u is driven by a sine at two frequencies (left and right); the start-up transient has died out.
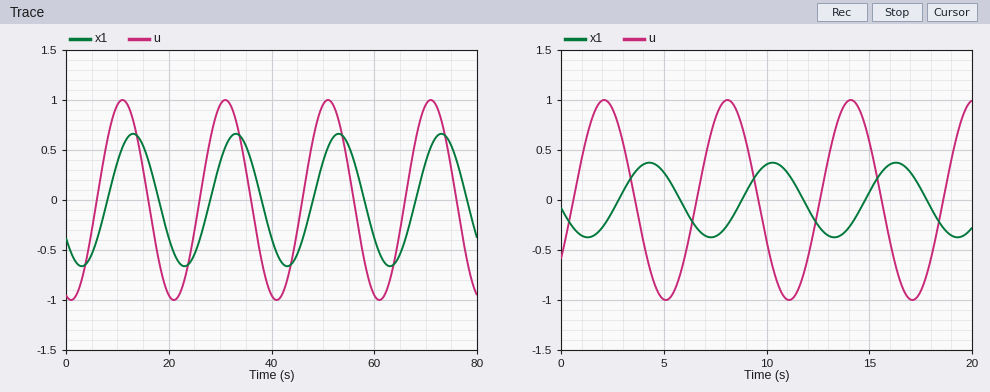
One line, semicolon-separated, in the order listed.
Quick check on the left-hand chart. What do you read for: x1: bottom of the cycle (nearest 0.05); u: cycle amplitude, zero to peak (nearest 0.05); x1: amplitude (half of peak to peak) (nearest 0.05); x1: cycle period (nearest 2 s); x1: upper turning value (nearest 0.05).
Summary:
-0.65; 1.00; 0.65; 20 s; 0.65
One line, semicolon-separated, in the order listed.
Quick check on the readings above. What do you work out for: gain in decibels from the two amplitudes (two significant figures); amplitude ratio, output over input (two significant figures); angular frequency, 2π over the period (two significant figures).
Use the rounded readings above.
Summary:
-3.7 dB; 0.65; 0.31 rad/s
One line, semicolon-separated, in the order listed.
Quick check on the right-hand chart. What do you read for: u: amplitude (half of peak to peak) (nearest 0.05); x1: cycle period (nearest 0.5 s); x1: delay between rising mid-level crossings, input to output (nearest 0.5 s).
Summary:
1.00; 6.0 s; 2.0 s
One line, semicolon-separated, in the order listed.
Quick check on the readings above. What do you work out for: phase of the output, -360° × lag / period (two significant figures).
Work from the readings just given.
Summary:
-120°
